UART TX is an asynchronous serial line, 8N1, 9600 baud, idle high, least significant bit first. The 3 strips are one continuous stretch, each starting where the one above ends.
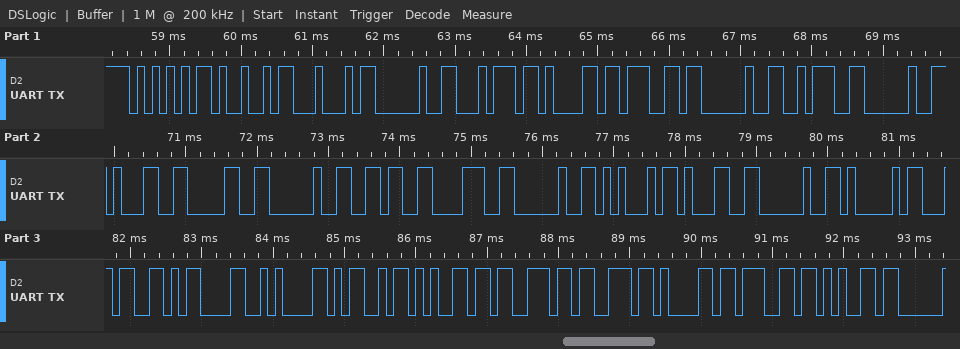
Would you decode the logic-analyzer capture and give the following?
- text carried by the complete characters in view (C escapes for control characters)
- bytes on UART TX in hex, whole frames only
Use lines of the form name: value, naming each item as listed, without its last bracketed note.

text carried by the complete characters in view: "UID tag : 10 68 E1 A4\r\nMessage"
bytes on UART TX in hex, whole frames only: 55 49 44 20 74 61 67 20 3A 20 31 30 20 36 38 20 45 31 20 41 34 0D 0A 4D 65 73 73 61 67 65
